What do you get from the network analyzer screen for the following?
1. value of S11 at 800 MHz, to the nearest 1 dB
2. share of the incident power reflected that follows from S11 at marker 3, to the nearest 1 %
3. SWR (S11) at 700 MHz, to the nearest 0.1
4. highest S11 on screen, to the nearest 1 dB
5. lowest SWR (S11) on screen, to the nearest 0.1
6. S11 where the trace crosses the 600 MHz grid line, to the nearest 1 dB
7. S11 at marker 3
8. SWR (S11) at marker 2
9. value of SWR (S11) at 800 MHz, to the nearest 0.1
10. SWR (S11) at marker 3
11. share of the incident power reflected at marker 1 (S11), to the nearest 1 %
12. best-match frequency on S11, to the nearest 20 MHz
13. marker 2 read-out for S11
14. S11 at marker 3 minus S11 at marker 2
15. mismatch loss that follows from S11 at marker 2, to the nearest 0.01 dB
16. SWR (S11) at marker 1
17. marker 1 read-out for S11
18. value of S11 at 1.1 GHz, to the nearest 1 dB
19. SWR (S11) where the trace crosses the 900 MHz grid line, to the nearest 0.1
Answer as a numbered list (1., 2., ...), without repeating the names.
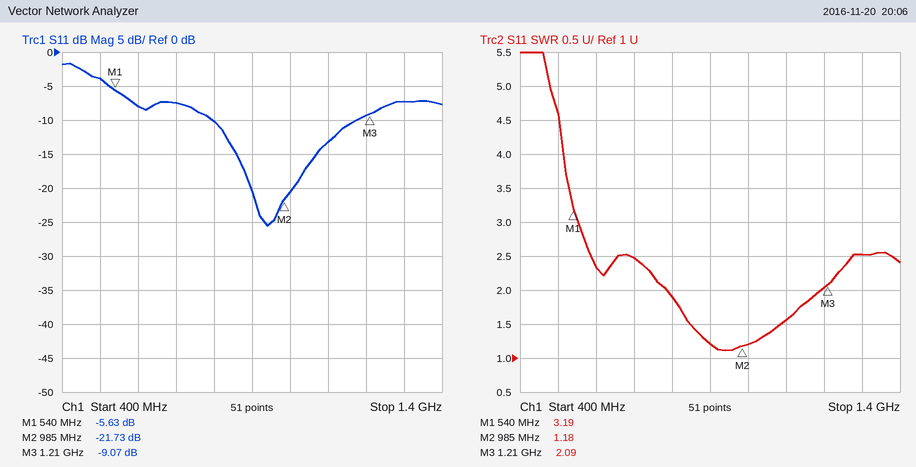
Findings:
1. -10 dB
2. 12 %
3. 2.5
4. -2 dB
5. 1.1
6. -8 dB
7. -9.07 dB
8. 1.18
9. 1.9
10. 2.09
11. 27 %
12. 940 MHz
13. -21.73 dB
14. 12.66 dB
15. 0.03 dB
16. 3.19
17. -5.63 dB
18. -13 dB
19. 1.2
